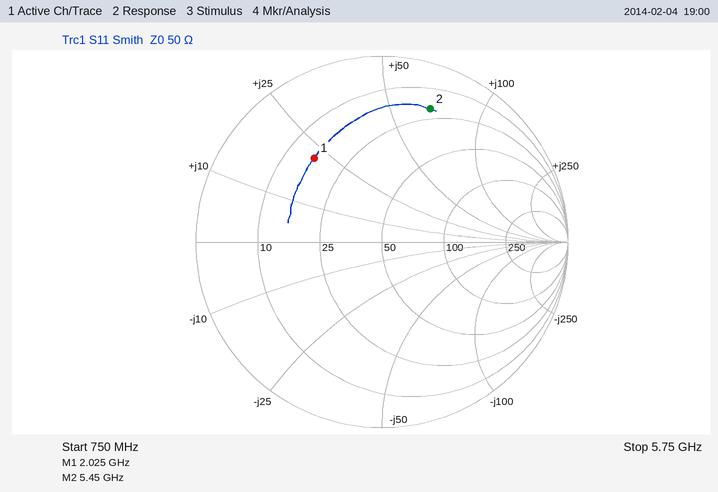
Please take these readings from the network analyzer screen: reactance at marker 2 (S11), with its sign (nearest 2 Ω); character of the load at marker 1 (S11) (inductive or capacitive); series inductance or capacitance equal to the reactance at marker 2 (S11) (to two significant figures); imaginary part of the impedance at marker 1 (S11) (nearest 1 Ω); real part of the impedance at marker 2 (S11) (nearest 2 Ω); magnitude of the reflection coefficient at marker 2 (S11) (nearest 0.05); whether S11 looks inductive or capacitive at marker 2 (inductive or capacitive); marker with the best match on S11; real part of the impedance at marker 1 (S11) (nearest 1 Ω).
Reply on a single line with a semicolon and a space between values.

+68 Ω; inductive; 2.0 nH; +22 Ω; 20 Ω; 0.75; inductive; marker 1; 16 Ω
